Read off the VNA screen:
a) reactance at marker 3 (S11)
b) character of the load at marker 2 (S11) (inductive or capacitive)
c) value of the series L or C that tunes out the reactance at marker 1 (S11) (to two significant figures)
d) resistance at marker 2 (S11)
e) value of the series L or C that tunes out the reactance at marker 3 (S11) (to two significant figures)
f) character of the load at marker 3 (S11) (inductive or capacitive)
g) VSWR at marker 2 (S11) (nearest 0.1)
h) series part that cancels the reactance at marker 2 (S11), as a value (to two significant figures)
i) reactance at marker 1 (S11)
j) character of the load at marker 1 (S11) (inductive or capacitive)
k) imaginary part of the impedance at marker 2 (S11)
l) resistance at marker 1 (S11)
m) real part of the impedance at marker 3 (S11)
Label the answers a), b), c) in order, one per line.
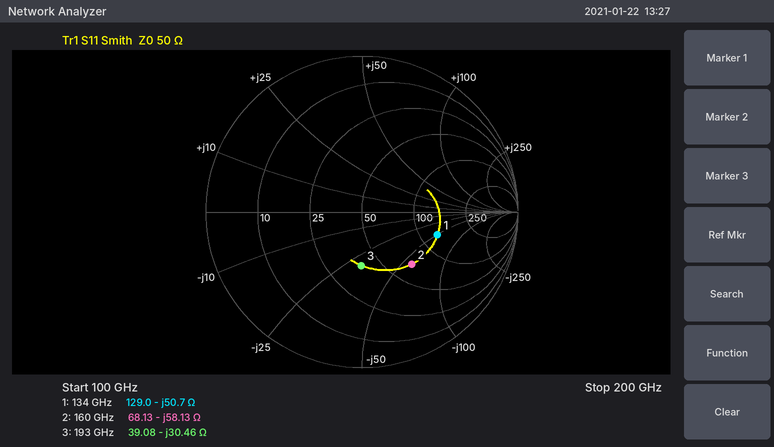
a) -30.46 Ω
b) capacitive
c) 60 pH
d) 68.13 Ω
e) 25 pH
f) capacitive
g) 2.7
h) 58 pH
i) -50.7 Ω
j) capacitive
k) -58.13 Ω
l) 129.0 Ω
m) 39.08 Ω
